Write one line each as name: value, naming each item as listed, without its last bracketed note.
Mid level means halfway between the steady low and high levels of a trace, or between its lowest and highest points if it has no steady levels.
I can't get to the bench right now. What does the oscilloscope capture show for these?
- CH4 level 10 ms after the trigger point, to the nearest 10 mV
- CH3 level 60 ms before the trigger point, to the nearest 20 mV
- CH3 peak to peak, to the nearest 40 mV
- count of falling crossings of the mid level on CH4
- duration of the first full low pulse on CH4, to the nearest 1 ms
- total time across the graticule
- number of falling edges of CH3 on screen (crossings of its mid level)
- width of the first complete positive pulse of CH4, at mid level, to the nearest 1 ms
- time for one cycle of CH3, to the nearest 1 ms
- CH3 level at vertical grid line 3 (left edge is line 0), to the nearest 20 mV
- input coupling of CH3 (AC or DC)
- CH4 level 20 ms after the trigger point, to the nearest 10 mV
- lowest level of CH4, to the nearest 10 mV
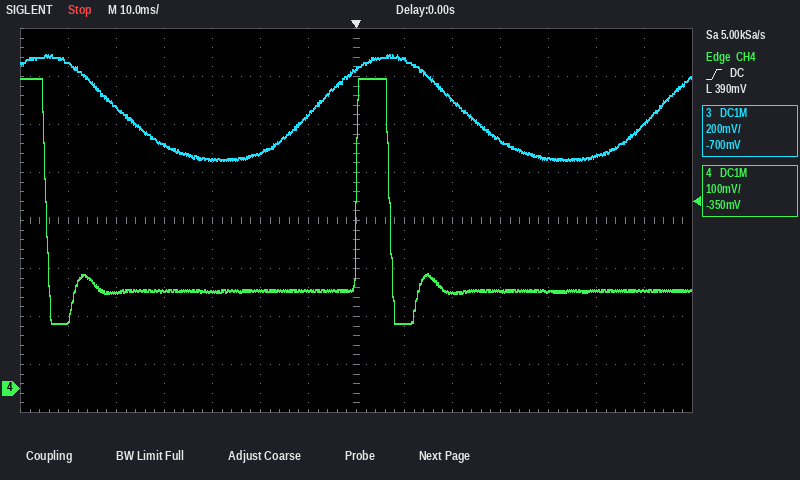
CH4 level 10 ms after the trigger point, to the nearest 10 mV: 140 mV
CH3 level 60 ms before the trigger point, to the nearest 20 mV: 1.36 V
CH3 peak to peak, to the nearest 40 mV: 440 mV
count of falling crossings of the mid level on CH4: 2
duration of the first full low pulse on CH4, to the nearest 1 ms: 65 ms
total time across the graticule: 140 ms
number of falling edges of CH3 on screen: 2
width of the first complete positive pulse of CH4, at mid level, to the nearest 1 ms: 7 ms
time for one cycle of CH3, to the nearest 1 ms: 72 ms
CH3 level at vertical grid line 3 (left edge is line 0), to the nearest 20 mV: 1.02 V
input coupling of CH3: DC
CH4 level 20 ms after the trigger point, to the nearest 10 mV: 200 mV
lowest level of CH4, to the nearest 10 mV: 140 mV
